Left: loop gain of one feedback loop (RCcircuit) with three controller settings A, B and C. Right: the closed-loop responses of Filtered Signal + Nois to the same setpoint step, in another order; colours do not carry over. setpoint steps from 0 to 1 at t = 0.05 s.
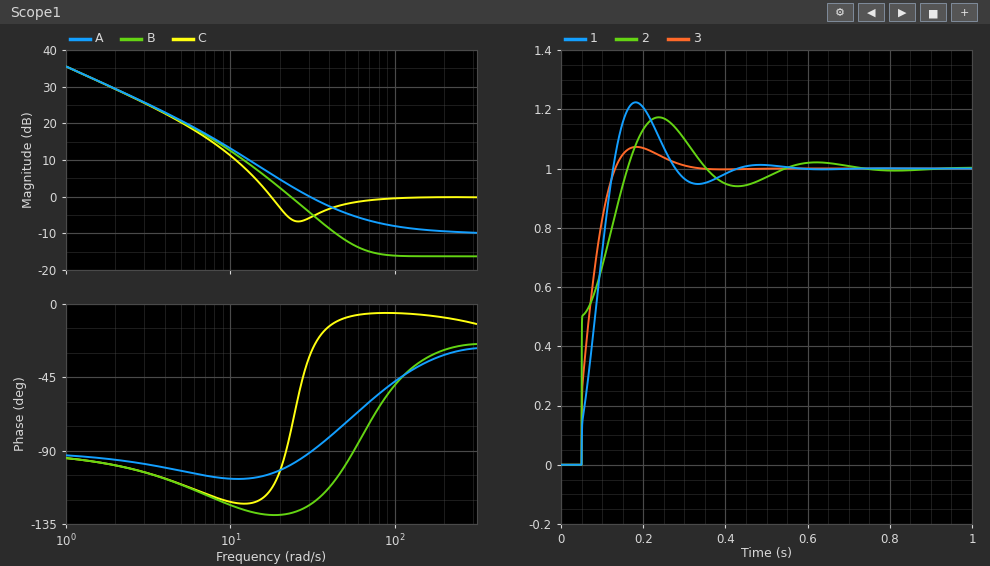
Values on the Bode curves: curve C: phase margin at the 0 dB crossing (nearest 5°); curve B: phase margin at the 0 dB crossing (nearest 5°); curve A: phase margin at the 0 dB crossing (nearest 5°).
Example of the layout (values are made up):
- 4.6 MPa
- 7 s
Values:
- 65°
- 50°
- 90°
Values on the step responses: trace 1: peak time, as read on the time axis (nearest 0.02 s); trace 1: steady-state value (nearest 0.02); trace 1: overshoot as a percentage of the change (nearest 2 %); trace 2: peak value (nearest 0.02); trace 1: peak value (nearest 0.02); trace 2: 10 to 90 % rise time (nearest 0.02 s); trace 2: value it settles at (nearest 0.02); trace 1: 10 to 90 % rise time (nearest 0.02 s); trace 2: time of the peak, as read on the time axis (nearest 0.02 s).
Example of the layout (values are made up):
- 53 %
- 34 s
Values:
- 0.18 s
- 1.00
- 22 %
- 1.18
- 1.22
- 0.10 s
- 1.00
- 0.06 s
- 0.24 s
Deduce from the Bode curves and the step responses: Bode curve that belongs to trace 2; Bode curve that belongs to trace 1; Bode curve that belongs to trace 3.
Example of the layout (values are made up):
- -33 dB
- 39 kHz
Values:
- C
- B
- A
